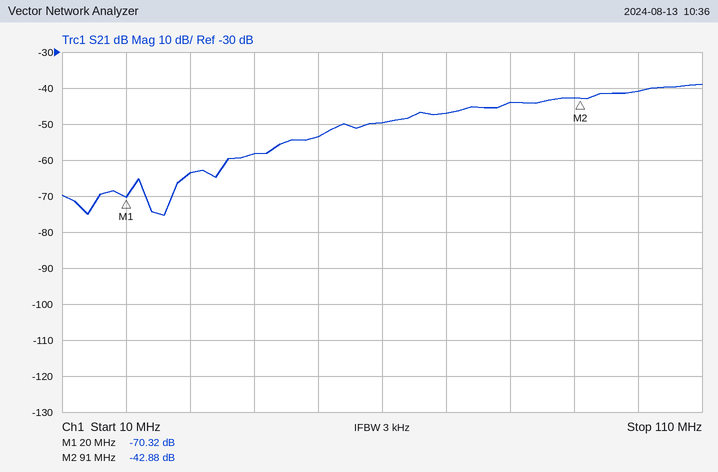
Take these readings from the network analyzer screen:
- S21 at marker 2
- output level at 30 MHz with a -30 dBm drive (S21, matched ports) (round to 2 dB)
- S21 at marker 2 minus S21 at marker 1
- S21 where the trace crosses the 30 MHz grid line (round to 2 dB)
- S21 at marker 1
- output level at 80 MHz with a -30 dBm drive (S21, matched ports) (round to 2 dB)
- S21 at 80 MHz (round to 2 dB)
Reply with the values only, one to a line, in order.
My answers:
-42.88 dB
-94 dBm
27.44 dB
-64 dB
-70.32 dB
-74 dBm
-44 dB
